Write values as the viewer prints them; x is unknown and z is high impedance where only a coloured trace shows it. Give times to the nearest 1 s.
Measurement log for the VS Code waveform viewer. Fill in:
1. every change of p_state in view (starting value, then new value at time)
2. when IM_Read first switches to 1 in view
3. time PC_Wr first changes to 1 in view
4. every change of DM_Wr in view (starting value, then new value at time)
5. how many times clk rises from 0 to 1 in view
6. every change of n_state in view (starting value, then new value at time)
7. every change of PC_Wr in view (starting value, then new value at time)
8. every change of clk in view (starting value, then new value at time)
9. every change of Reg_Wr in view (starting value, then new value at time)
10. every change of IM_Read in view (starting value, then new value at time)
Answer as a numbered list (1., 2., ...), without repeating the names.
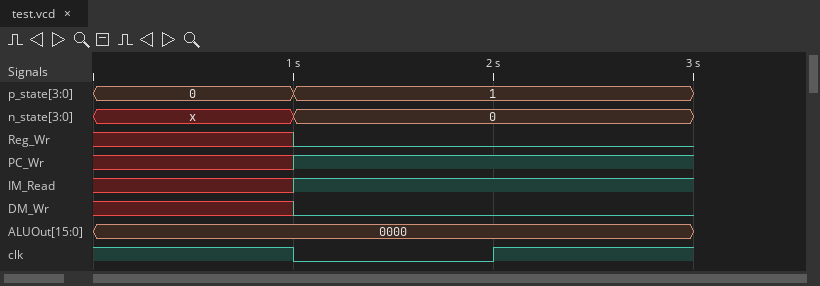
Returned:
1. 0, 1 at 1 s
2. 1 s
3. 1 s
4. x, 0 at 1 s
5. 1
6. x, 0 at 1 s
7. x, 1 at 1 s
8. 1, 0 at 1 s, 1 at 2 s
9. x, 0 at 1 s
10. x, 1 at 1 s
